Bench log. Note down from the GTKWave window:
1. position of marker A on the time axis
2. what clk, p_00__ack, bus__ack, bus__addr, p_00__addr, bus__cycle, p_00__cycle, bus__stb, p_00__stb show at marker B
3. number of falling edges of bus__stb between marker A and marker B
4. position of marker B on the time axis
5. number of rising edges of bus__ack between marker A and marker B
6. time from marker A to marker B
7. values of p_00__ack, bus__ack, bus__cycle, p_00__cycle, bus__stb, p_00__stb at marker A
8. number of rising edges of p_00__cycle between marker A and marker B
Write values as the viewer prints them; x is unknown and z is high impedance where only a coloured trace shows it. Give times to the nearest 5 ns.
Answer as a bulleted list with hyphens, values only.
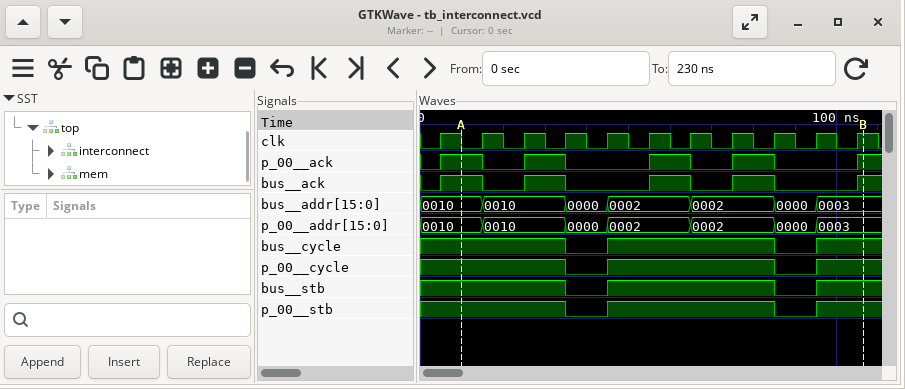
- 10 ns
- clk=1, p_00__ack=1, bus__ack=1, bus__addr=0003, p_00__addr=0003, bus__cycle=1, p_00__cycle=1, bus__stb=1, p_00__stb=1
- 2
- 105 ns
- 4
- 95 ns
- p_00__ack=1, bus__ack=1, bus__cycle=1, p_00__cycle=1, bus__stb=1, p_00__stb=1
- 2
